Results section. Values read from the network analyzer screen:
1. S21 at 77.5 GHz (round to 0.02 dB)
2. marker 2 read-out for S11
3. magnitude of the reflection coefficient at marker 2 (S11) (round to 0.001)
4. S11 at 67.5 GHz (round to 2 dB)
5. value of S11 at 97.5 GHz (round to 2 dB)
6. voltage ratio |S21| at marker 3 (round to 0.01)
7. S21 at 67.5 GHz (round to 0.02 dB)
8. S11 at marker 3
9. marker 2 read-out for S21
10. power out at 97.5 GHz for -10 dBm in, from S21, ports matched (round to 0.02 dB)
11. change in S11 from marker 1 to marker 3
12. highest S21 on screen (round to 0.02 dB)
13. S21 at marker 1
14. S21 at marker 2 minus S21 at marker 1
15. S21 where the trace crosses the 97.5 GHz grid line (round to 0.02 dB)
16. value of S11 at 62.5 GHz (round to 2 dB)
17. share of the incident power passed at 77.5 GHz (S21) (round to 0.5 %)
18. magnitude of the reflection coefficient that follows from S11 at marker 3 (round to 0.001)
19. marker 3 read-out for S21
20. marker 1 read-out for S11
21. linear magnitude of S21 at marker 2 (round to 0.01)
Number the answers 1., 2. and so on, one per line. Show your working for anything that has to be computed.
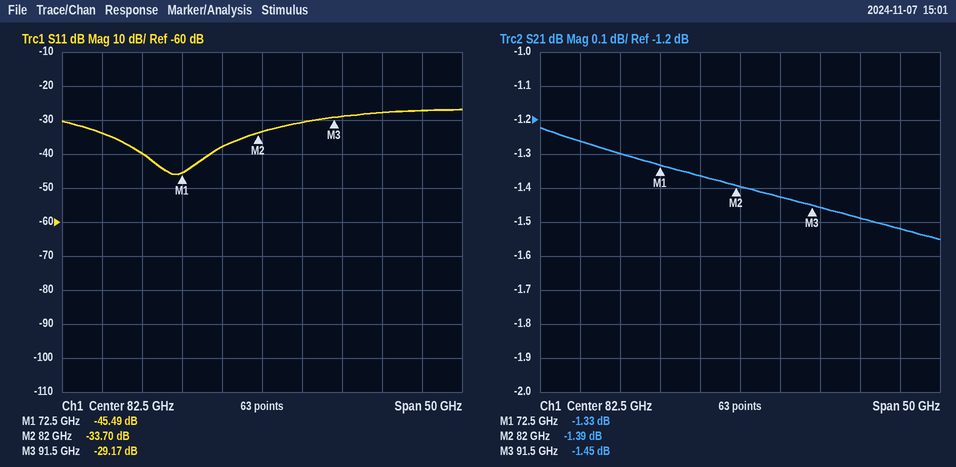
1. -1.36 dB
2. -33.70 dB
3. 10^(-33.7/20) ≈ 0.021
4. -40 dB
5. -28 dB
6. 10^(-1.45/20) ≈ 0.85
7. -1.30 dB
8. -29.17 dB
9. -1.39 dB
10. -10 dBm + (-1.48 dB) = -11.48 dBm
11. -29.17 − (-45.49) = 16.32 dB
12. -1.22 dB
13. -1.33 dB
14. -1.39 − (-1.33) = -0.06 dB
15. -1.48 dB
16. -34 dB
17. 10^(-1.36/10) ≈ 73.1 %, so 73.0 % to the nearest 0.5 %
18. 10^(-29.17/20) ≈ 0.035
19. -1.45 dB
20. -45.49 dB
21. 10^(-1.39/20) ≈ 0.85
